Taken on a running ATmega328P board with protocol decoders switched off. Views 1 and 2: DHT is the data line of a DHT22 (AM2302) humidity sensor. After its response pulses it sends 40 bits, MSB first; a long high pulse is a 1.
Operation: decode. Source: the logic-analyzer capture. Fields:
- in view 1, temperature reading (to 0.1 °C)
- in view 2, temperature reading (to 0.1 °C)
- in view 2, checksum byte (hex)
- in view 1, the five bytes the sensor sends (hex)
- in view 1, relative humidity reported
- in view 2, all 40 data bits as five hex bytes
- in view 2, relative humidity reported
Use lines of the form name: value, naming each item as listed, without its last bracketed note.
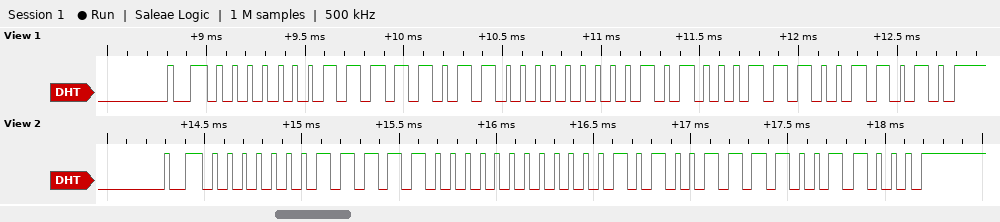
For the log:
in view 1, temperature reading: 16.3 °C
in view 2, temperature reading: 16.7 °C
in view 2, checksum byte: 0x98
in view 1, the five bytes the sensor sends: 01 F6 00 A3 9A
in view 1, relative humidity reported: 50.2 %
in view 2, all 40 data bits as five hex bytes: 01 F0 00 A7 98
in view 2, relative humidity reported: 49.6 %
